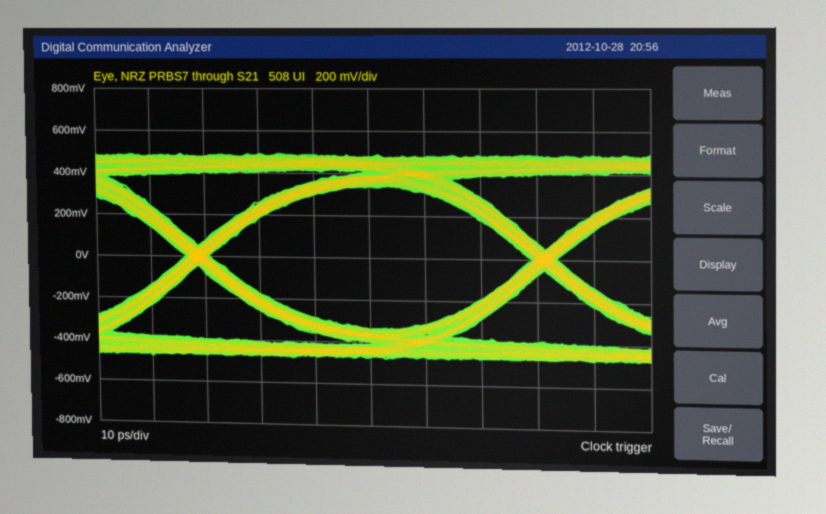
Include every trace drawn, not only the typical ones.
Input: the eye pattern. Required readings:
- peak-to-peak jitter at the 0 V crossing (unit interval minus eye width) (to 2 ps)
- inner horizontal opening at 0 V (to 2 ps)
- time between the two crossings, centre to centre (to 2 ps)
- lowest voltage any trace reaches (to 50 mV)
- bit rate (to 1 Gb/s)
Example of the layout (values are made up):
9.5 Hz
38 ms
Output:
4 ps
58 ps
62 ps
-500 mV
16 Gb/s
